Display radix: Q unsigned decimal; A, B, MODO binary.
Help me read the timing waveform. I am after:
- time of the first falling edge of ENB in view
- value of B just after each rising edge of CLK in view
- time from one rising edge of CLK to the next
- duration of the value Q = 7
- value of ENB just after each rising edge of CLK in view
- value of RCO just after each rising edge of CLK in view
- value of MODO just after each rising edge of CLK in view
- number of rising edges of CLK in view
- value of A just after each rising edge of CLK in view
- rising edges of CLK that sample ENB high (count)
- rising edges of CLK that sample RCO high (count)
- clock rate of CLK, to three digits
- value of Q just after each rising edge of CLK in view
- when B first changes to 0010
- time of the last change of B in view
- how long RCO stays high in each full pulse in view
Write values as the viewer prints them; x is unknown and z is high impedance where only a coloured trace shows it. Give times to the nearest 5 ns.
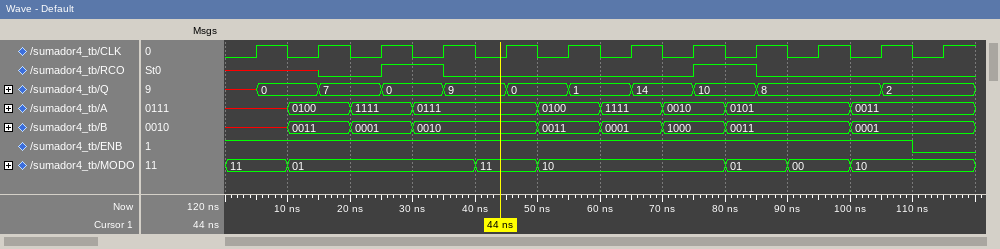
110 ns
x, 0011, 0001, 0010, 0010, 0011, 0001, 1000, 0011, 0011, 0001, 0001
10 ns
10 ns
1 1 1 1 1 1 1 1 1 1 1 0
x 0 1 0 0 0 0 1 0 0 0 0
11, 01, 01, 01, 11, 10, 10, 10, 01, 00, 10, 10
12
x, 0100, 1111, 0111, 0111, 0100, 1111, 0010, 0101, 0101, 0011, 0011
11
2
100 MHz
0, 7, 0, 9, 0, 1, 14, 10, 8, 8, 2, 2
30 ns
100 ns
10 ns, 10 ns
